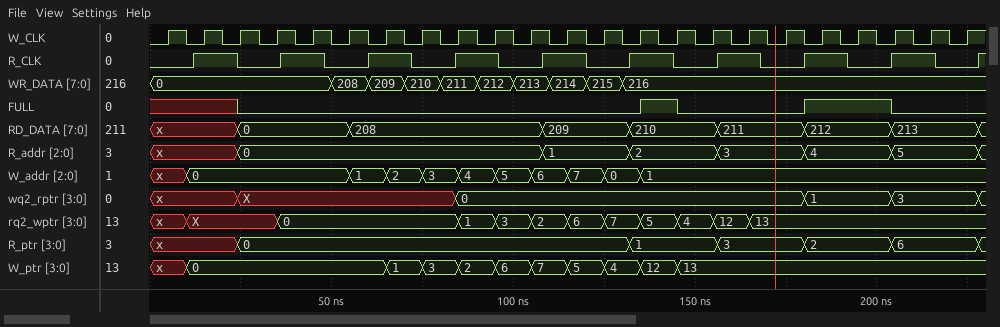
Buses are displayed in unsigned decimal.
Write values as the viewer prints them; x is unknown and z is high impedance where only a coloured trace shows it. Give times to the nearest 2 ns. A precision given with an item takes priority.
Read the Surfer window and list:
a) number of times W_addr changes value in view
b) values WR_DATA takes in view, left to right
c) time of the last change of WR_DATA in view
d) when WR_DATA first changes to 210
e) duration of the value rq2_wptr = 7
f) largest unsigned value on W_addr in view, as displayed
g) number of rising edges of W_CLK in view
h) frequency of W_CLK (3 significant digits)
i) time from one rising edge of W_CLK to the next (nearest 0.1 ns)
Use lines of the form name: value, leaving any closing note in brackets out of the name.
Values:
number of times W_addr changes value in view: 10
values WR_DATA takes in view, left to right: 0, 208, 209, 210, 211, 212, 213, 214, 215, 216
time of the last change of WR_DATA in view: 130 ns
when WR_DATA first changes to 210: 70 ns
duration of the value rq2_wptr = 7: 10 ns
largest unsigned value on W_addr in view, as displayed: 7
number of rising edges of W_CLK in view: 23
frequency of W_CLK: 100 MHz
time from one rising edge of W_CLK to the next: 10 ns
